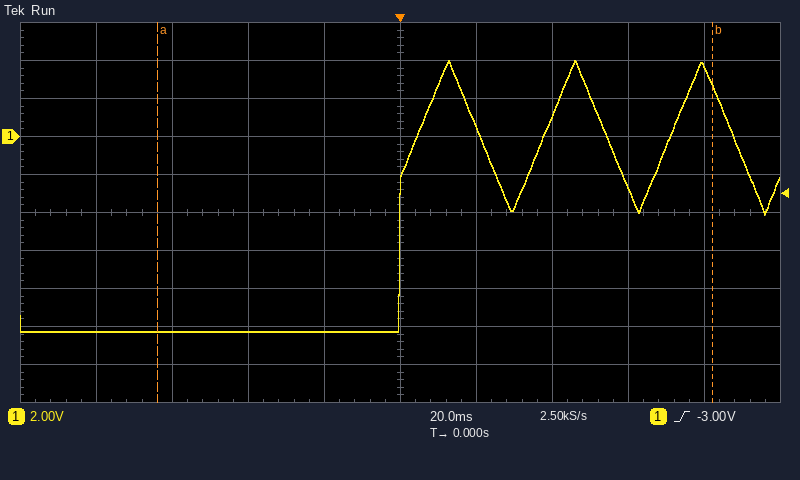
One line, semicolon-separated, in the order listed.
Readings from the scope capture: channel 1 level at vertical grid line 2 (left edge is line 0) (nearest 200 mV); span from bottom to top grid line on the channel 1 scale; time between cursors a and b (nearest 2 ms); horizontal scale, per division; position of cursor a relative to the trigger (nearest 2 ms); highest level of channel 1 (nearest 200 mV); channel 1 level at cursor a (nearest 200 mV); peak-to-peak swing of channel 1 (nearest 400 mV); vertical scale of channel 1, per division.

-10.2 V; 20 V; 146 ms; 20 ms; -64 ms; 4.0 V; -10.2 V; 14.4 V; 2 V
